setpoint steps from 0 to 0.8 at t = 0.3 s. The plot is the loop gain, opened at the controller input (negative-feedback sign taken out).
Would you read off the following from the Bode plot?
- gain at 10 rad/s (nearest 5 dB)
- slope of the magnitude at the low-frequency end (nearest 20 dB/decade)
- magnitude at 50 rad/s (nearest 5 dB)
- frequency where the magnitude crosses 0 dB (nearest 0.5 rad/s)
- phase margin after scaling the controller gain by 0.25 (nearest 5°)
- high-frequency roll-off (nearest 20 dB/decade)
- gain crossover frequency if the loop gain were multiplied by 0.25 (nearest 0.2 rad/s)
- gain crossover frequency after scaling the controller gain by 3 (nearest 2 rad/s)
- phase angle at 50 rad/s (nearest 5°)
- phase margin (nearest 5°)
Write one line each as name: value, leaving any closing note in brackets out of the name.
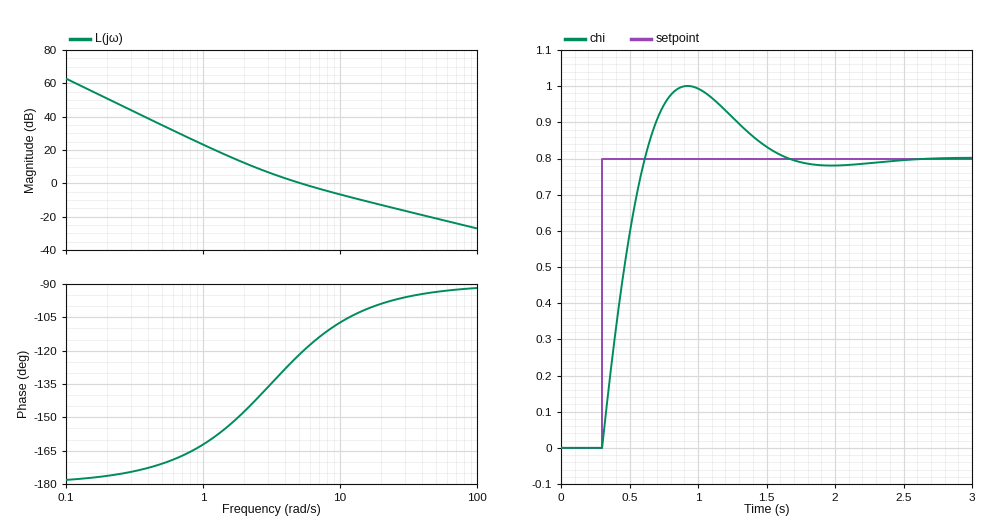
gain at 10 rad/s: -5 dB
slope of the magnitude at the low-frequency end: -40 dB/decade
magnitude at 50 rad/s: -20 dB
frequency where the magnitude crosses 0 dB: 5.0 rad/s
phase margin after scaling the controller gain by 0.25: 35°
high-frequency roll-off: -20 dB/decade
gain crossover frequency if the loop gain were multiplied by 0.25: 2.0 rad/s
gain crossover frequency after scaling the controller gain by 3: 14 rad/s
phase angle at 50 rad/s: -95°
phase margin: 60°
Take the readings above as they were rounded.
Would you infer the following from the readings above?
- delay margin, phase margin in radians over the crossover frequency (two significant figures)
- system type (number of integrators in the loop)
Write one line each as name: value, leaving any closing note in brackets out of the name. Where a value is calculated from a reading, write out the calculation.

delay margin, phase margin in radians over the crossover frequency: 60 × π / 180 / 5 = 0.21 s
system type: 2
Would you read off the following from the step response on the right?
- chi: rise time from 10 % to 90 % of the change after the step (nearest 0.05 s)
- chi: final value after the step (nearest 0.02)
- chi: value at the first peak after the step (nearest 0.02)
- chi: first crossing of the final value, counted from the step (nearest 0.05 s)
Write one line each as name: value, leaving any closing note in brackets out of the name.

chi: rise time from 10 % to 90 % of the change after the step: 0.25 s
chi: final value after the step: 0.80
chi: value at the first peak after the step: 1.00
chi: first crossing of the final value, counted from the step: 0.30 s
